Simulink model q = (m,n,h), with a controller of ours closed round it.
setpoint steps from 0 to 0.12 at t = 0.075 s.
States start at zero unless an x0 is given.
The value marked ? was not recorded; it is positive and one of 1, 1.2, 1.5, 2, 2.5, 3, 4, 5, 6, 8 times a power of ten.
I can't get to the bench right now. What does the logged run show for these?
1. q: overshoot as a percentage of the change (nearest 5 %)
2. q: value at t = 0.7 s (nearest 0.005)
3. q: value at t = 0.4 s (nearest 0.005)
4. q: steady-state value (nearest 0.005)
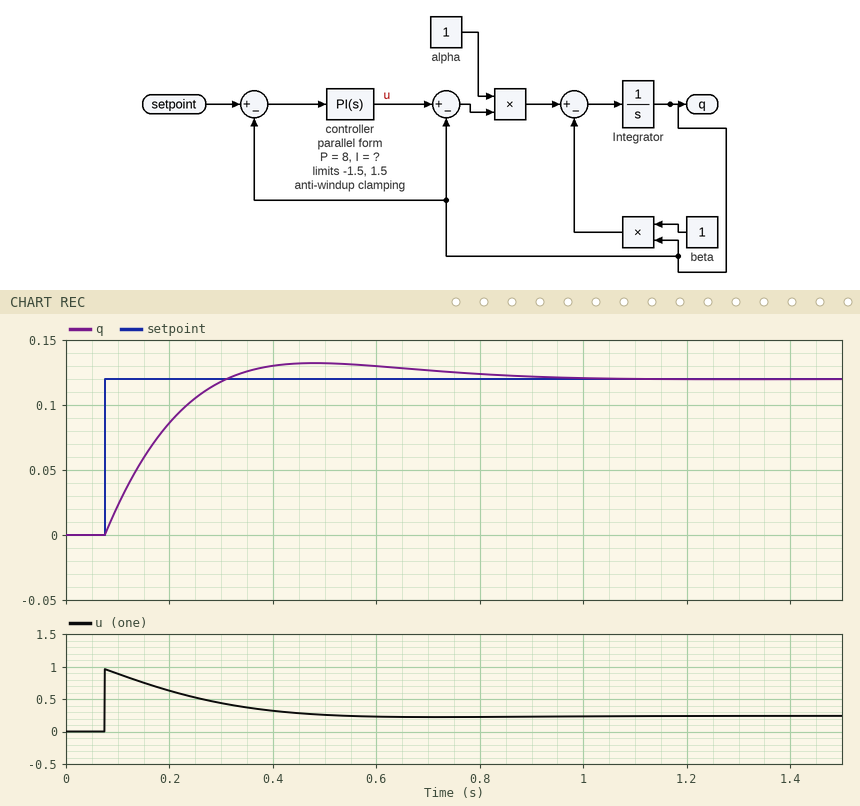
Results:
10 %
0.125
0.130
0.120
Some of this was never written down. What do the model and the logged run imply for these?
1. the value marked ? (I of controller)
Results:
40
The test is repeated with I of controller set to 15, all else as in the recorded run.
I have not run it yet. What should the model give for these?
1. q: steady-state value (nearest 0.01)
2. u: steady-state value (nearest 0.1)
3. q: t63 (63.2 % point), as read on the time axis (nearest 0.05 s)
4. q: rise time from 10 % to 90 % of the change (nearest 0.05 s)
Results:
0.12
0.2
0.20 s
0.30 s
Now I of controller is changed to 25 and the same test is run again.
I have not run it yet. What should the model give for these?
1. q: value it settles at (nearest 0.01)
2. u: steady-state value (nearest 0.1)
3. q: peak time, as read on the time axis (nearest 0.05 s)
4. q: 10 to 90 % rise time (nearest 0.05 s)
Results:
0.12
0.2
0.60 s
0.20 s
